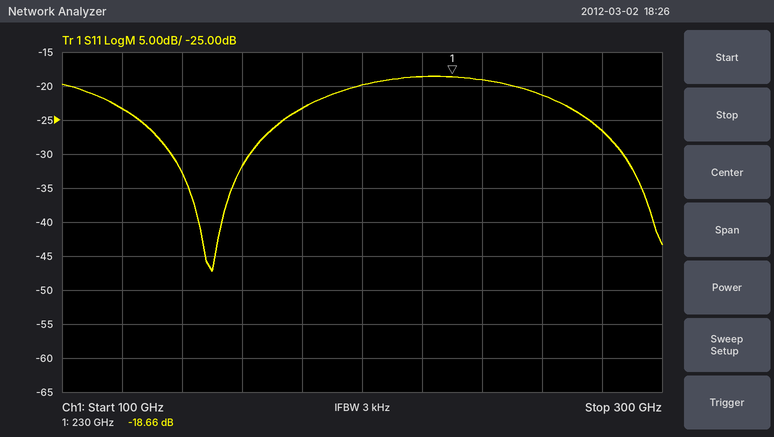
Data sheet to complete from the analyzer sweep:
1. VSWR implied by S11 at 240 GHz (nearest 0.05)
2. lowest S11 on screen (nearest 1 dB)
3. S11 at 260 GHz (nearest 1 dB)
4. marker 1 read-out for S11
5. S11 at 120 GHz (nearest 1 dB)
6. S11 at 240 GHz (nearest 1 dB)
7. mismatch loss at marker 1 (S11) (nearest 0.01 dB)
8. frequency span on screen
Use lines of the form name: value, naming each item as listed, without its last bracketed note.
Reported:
VSWR implied by S11 at 240 GHz: 1.25
lowest S11 on screen: -47 dB
S11 at 260 GHz: -21 dB
marker 1 read-out for S11: -18.66 dB
S11 at 120 GHz: -23 dB
S11 at 240 GHz: -19 dB
mismatch loss at marker 1 (S11): 0.06 dB
frequency span on screen: 200 GHz
